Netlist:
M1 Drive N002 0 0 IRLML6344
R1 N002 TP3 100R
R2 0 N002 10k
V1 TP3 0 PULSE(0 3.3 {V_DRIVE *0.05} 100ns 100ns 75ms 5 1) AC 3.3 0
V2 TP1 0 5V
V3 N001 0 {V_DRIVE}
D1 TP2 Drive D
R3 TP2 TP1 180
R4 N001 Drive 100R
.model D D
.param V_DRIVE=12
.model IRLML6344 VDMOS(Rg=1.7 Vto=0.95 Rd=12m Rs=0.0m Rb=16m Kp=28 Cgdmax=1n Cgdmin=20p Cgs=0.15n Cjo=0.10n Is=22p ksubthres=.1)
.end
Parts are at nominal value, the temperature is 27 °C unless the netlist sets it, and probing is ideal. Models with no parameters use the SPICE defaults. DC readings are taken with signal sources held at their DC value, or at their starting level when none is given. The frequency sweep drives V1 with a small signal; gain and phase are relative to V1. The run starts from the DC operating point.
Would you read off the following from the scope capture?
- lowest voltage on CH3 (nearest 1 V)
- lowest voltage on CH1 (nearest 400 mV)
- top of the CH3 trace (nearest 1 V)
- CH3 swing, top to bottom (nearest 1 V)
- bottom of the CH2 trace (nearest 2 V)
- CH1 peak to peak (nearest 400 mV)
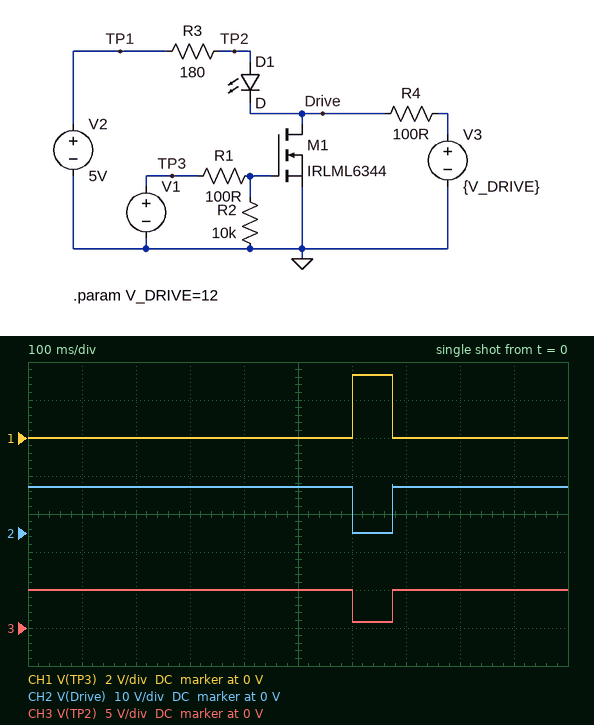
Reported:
1 V
0 V
5 V
4 V
0 V
3.2 V
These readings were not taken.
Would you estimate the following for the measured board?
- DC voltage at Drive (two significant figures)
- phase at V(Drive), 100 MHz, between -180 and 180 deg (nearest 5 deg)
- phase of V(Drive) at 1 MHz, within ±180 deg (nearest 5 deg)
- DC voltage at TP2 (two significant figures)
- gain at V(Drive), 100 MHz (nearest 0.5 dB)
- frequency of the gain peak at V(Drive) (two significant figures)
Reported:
12 V
-70 deg
80 deg
5.0 V
-24.5 dB
14 MHz
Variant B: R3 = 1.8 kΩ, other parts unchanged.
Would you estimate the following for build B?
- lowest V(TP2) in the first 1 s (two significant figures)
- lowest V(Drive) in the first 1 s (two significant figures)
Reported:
680 mV
3.3 mV
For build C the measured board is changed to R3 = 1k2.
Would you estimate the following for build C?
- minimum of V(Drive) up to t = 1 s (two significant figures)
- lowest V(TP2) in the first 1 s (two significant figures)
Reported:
3.4 mV
690 mV
